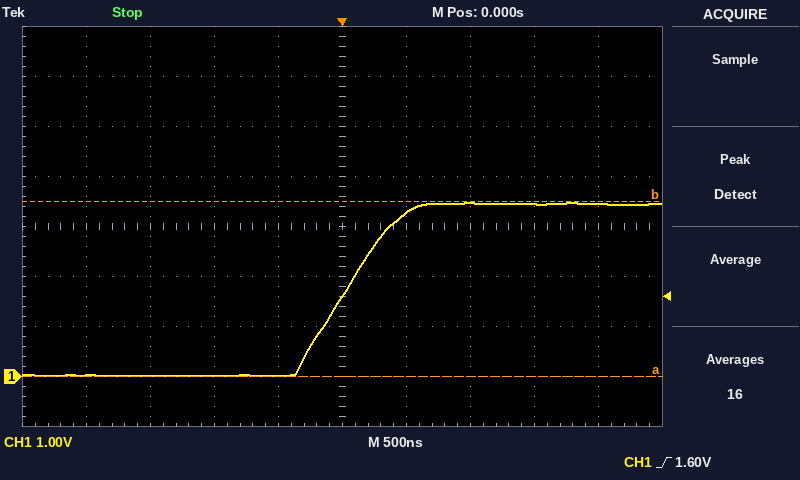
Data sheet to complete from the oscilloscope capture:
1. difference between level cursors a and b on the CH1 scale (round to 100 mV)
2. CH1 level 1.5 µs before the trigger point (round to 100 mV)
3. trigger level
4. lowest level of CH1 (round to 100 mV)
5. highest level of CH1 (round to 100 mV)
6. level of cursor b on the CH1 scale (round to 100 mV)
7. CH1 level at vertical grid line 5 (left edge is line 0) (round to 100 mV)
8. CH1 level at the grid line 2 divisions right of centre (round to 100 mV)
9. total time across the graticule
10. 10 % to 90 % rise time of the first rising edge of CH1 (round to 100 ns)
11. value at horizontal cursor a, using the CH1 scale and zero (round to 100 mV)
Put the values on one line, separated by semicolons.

3.5 V; 0.0 V; 1.60 V; 0.0 V; 3.5 V; 3.5 V; 1.6 V; 3.5 V; 5 µs; 700 ns; 0.0 V
